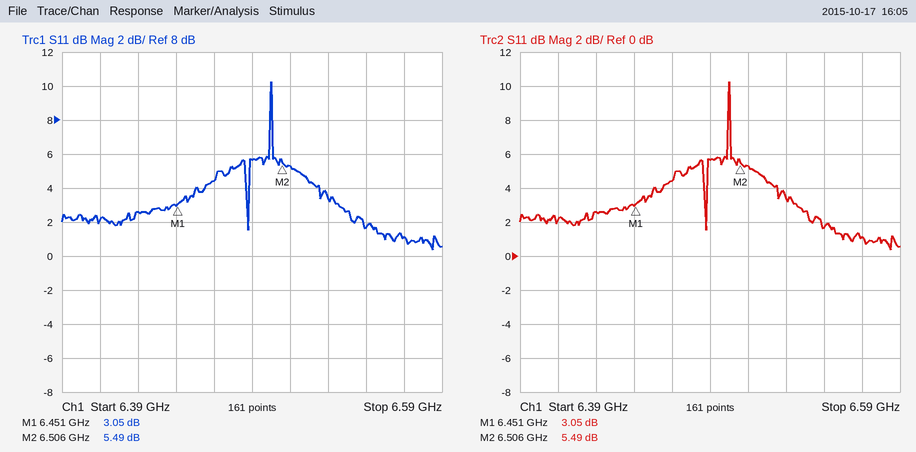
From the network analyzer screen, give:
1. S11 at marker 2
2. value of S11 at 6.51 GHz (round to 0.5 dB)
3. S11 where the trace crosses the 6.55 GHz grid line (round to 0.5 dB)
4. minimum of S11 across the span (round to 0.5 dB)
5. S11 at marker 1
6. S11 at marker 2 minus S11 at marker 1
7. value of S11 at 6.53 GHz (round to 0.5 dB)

5.49 dB
5.5 dB
1.5 dB
0.5 dB
3.05 dB
2.44 dB
3.5 dB
